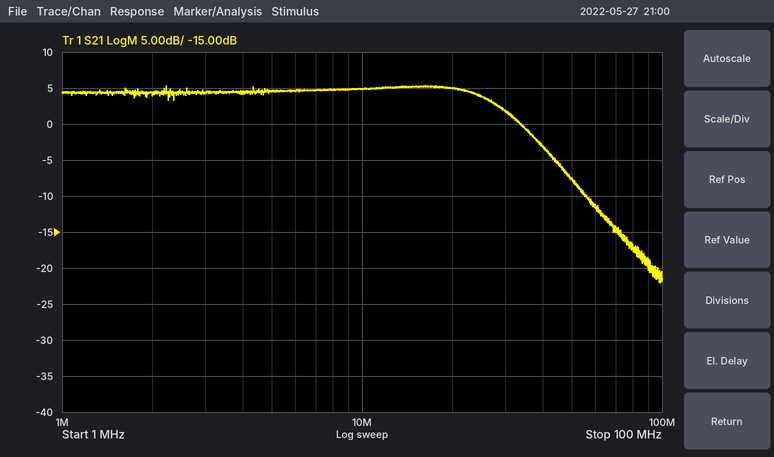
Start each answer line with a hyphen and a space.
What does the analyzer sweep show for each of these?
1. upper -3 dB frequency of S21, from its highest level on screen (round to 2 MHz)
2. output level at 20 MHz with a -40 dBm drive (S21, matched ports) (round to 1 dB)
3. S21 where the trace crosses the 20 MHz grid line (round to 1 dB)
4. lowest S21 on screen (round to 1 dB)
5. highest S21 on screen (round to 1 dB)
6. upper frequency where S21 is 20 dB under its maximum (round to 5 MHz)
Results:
- 28 MHz
- -35 dBm
- 5 dB
- -22 dB
- 5 dB
- 70 MHz
